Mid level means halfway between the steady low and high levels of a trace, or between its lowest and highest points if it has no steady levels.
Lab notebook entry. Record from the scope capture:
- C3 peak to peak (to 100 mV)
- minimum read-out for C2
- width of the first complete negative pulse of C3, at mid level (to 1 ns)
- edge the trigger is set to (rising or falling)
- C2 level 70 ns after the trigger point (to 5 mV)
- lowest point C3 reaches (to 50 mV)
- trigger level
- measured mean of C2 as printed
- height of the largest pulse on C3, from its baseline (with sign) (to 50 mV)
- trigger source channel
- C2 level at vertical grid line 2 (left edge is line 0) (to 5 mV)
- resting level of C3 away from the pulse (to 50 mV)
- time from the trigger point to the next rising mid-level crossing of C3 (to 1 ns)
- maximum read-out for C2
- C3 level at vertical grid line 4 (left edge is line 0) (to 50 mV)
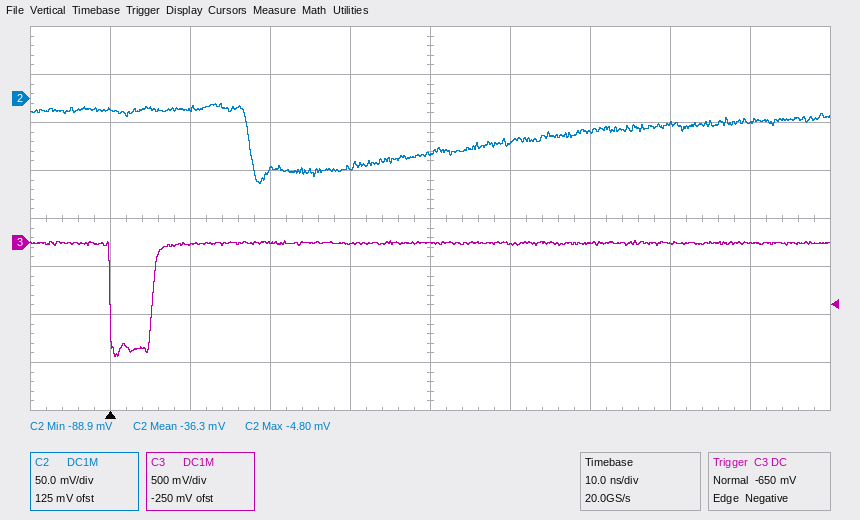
1.20 V
-88.9 mV
5 ns
falling
-25 mV
-1.20 V
-650 mV
-36.3 mV
-1.20 V
C3
-10 mV
0 mV
5 ns
-4.80 mV
0 mV
